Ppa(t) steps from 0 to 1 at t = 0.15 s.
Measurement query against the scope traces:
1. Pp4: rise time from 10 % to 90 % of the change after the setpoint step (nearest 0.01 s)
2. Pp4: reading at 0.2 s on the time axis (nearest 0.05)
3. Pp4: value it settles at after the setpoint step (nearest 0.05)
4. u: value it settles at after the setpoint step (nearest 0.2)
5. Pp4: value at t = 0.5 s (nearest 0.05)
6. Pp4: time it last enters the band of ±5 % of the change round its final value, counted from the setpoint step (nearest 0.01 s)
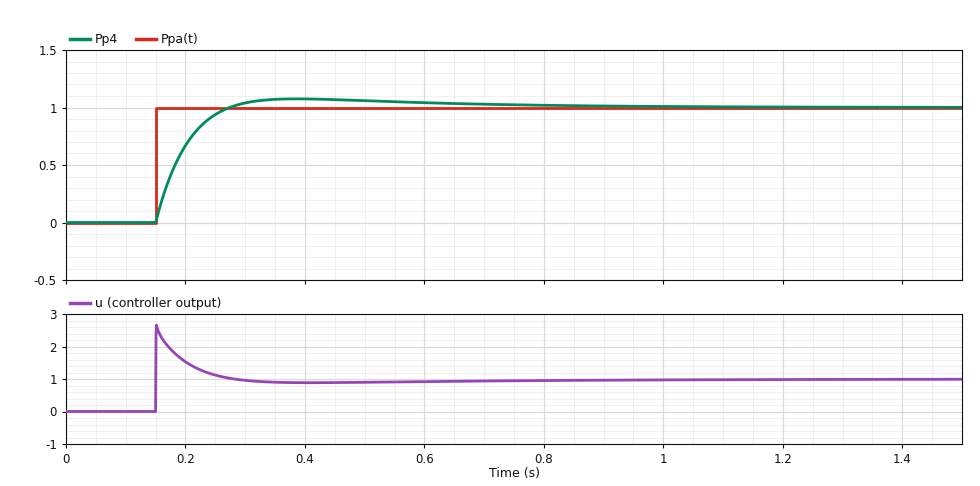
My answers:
0.08 s
0.65
1.00
1.0
1.05
0.40 s
